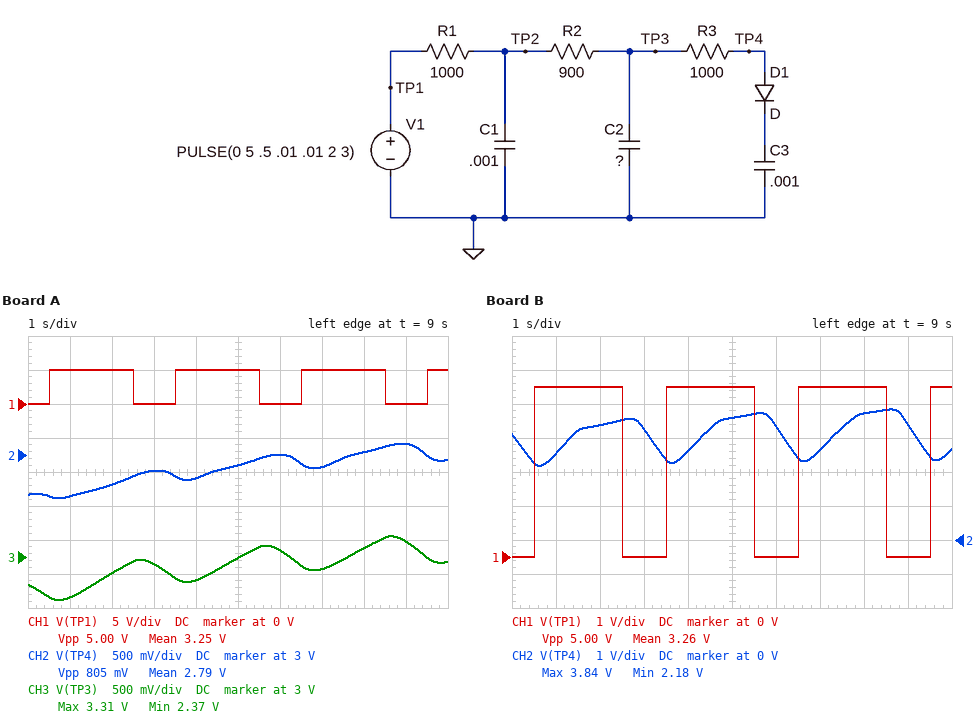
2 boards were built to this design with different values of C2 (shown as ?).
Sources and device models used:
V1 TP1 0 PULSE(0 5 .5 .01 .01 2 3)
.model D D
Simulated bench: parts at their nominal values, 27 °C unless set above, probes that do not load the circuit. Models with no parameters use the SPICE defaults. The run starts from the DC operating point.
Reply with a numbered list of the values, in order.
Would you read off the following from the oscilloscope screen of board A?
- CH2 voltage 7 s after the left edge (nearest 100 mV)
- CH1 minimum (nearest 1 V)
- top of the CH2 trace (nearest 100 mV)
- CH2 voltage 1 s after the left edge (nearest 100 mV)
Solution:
1. 2.8 V
2. 0 V
3. 3.2 V
4. 2.4 V
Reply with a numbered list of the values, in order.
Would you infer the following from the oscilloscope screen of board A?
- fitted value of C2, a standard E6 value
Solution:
1. 2.2 mF
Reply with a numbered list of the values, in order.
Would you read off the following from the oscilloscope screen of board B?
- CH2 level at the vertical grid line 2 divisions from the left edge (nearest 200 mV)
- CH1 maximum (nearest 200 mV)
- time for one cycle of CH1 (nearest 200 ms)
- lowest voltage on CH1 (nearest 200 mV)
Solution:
1. 3.4 V
2. 5.0 V
3. 3.0 s
4. 0 V
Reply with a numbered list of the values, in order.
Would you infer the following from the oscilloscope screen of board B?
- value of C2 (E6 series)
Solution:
1. 330 µF
